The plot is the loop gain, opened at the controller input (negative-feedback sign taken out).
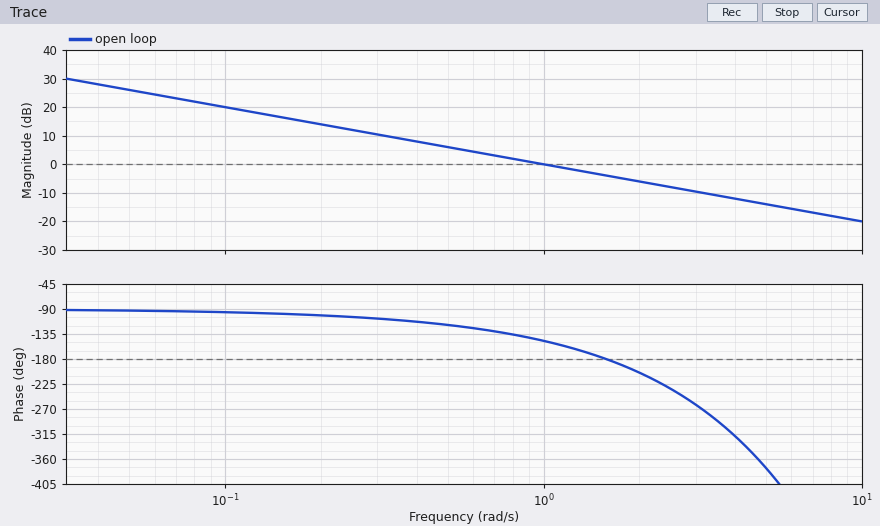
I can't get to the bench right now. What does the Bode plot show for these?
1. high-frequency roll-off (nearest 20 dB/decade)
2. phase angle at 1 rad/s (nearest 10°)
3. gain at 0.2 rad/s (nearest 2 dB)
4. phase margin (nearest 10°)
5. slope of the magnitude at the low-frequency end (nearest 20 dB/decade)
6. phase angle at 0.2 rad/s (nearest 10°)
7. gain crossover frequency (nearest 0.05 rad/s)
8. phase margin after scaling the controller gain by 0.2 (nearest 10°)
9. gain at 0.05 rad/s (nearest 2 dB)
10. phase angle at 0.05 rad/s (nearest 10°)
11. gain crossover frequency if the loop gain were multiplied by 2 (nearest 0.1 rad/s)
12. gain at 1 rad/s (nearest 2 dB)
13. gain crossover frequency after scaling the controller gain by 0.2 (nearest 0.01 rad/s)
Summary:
-20 dB/decade
-150°
14 dB
30°
-20 dB/decade
-100°
1.00 rad/s
80°
26 dB
-90°
2.0 rad/s
0 dB
0.20 rad/s
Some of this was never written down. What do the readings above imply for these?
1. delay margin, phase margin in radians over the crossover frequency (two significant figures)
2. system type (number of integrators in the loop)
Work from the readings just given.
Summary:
0.52 s
1
